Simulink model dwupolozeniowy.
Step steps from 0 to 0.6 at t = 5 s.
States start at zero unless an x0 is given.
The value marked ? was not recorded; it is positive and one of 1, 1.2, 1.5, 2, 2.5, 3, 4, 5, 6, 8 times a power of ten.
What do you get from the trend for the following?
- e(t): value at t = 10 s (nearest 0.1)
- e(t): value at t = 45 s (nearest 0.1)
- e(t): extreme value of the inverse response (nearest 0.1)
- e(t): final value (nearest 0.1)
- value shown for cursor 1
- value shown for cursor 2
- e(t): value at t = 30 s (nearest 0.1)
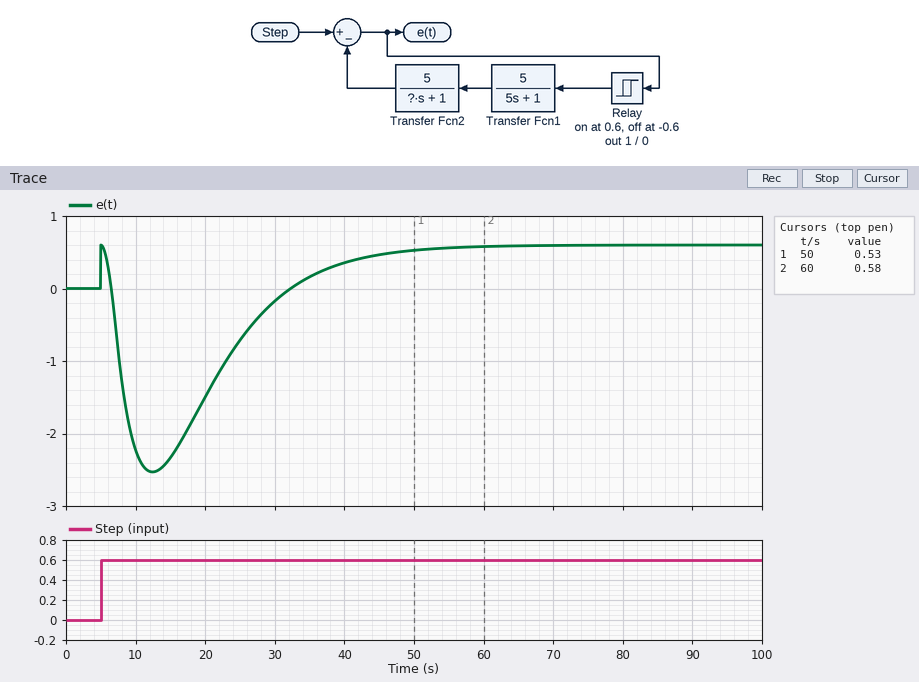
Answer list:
-2.2
0.5
-2.5
0.6
0.53
0.58
-0.2
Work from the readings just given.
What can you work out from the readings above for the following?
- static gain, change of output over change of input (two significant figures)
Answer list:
1.0
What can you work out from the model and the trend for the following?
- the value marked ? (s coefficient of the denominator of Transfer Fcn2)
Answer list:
8
